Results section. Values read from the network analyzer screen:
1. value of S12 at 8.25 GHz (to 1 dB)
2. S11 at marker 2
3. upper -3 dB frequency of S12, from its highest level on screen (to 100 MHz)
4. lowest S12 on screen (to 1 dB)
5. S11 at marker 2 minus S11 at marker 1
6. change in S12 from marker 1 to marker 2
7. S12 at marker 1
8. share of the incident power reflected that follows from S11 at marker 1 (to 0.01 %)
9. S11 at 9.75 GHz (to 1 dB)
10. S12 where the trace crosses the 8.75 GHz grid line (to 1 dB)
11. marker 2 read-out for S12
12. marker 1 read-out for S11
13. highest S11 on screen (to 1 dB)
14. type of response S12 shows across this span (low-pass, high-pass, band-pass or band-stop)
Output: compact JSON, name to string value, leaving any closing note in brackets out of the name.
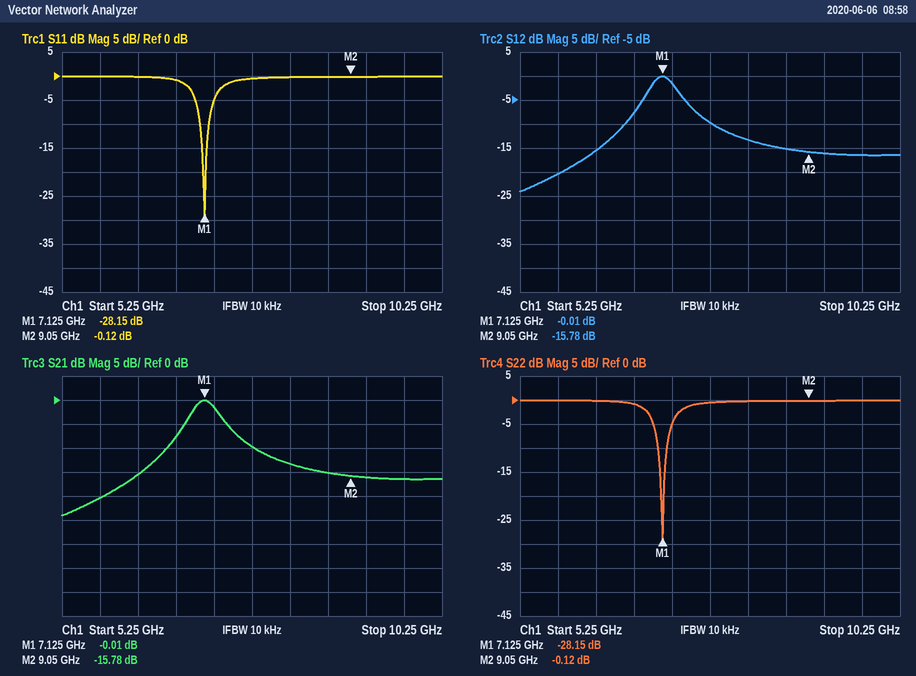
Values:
{"value of S12 at 8.25 GHz": "-13 dB", "S11 at marker 2": "-0.12 dB", "upper -3 dB frequency of S12, from its highest level on screen": "7.3 GHz", "lowest S12 on screen": "-24 dB", "S11 at marker 2 minus S11 at marker 1": "28.03 dB", "change in S12 from marker 1 to marker 2": "-15.77 dB", "S12 at marker 1": "-0.01 dB", "share of the incident power reflected that follows from S11 at marker 1": "0.15 %", "S11 at 9.75 GHz": "0 dB", "S12 where the trace crosses the 8.75 GHz grid line": "-15 dB", "marker 2 read-out for S12": "-15.78 dB", "marker 1 read-out for S11": "-28.15 dB", "highest S11 on screen": "0 dB", "type of response S12 shows across this span": "band-pass"}
